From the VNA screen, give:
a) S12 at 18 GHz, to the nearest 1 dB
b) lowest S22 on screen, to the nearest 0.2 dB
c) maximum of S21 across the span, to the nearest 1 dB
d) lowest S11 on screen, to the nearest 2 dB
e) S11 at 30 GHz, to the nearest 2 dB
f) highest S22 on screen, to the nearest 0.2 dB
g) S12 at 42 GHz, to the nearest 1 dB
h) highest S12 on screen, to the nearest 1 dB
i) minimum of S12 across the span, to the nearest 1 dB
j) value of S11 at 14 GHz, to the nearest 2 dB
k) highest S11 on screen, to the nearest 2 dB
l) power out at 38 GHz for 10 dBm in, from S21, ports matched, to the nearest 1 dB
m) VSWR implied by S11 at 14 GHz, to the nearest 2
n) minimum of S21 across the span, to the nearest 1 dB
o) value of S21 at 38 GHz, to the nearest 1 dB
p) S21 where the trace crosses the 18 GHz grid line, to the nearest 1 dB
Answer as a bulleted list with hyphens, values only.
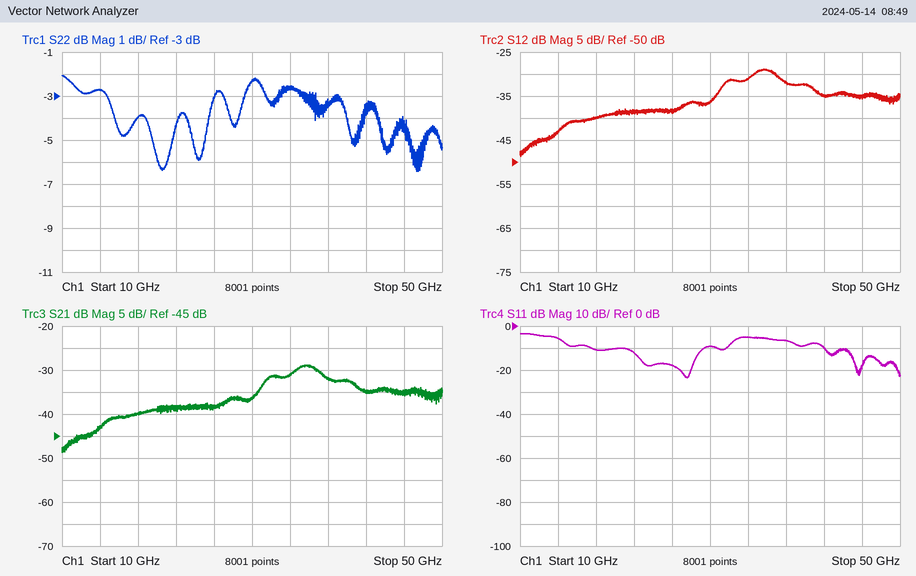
- -40 dB
- -6.4 dB
- -29 dB
- -24 dB
- -10 dB
- -2.0 dB
- -35 dB
- -29 dB
- -49 dB
- -6 dB
- -4 dB
- -22 dBm
- 4
- -49 dB
- -32 dB
- -40 dB
